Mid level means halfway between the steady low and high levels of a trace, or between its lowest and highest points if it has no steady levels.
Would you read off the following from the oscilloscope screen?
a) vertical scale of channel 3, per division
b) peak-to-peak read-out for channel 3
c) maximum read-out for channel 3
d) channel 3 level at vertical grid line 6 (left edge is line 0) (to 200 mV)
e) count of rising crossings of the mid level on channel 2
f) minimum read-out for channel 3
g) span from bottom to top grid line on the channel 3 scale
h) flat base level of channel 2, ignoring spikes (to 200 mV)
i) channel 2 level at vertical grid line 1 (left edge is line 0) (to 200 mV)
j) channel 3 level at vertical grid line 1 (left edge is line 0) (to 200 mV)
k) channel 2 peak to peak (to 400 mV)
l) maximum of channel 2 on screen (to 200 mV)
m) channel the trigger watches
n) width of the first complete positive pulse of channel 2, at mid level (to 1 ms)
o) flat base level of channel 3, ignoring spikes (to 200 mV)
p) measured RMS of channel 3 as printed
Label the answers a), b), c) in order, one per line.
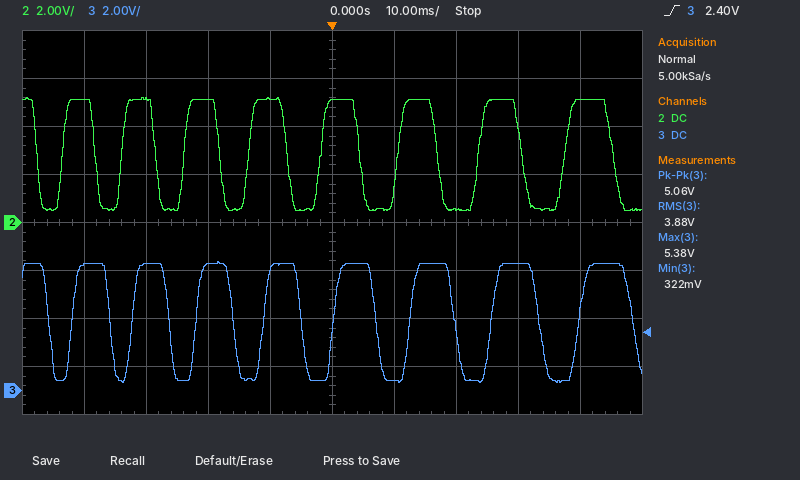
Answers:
a) 2 V
b) 5.06 V
c) 5.38 V
d) 400 mV
e) 8
f) 322 mV
g) 16 V
h) 600 mV
i) 5.2 V
j) 5.2 V
k) 4.8 V
l) 5.2 V
m) channel 3
n) 5 ms
o) 400 mV
p) 3.88 V
